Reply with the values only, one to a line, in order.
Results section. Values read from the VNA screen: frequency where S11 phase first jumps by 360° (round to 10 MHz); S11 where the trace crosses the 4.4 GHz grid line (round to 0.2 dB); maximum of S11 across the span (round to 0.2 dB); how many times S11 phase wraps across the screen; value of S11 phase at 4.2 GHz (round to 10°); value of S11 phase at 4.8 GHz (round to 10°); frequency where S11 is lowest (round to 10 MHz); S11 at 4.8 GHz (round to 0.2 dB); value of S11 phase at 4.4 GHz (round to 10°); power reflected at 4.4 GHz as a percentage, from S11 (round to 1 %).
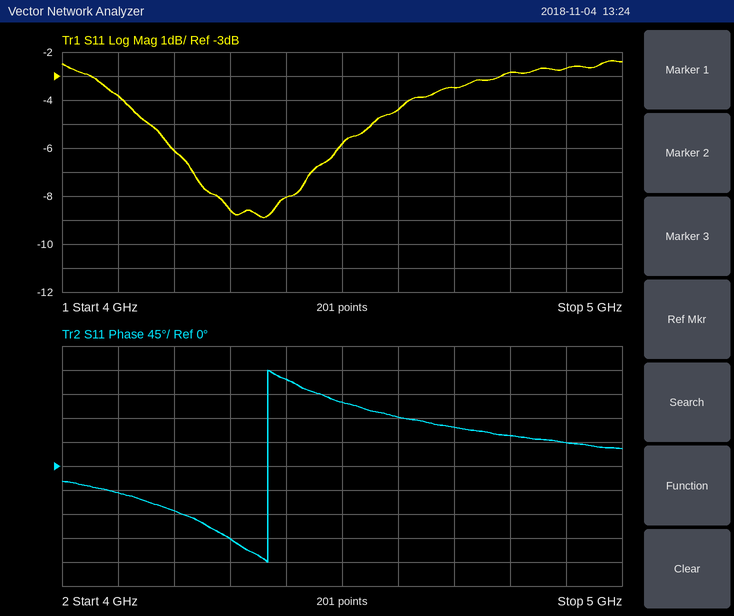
4.37 GHz
-8.0 dB
-2.4 dB
1
-80°
60°
4.36 GHz
-2.8 dB
160°
16 %
